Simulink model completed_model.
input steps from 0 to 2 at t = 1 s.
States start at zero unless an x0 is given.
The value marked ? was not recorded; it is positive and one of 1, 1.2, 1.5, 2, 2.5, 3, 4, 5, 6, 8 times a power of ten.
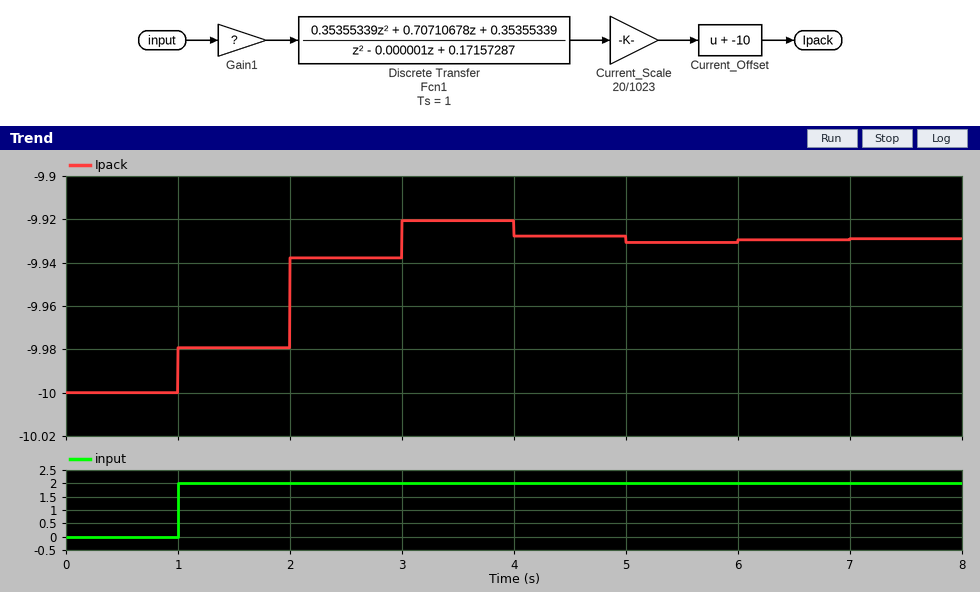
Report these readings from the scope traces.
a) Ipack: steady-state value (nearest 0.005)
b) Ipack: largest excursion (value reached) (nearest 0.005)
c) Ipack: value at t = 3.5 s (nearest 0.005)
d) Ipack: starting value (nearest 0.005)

-9.930
-9.920
-9.920
-10.000
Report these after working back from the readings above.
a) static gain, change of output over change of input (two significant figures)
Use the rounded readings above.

0.035
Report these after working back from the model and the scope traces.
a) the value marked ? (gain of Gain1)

1.5
